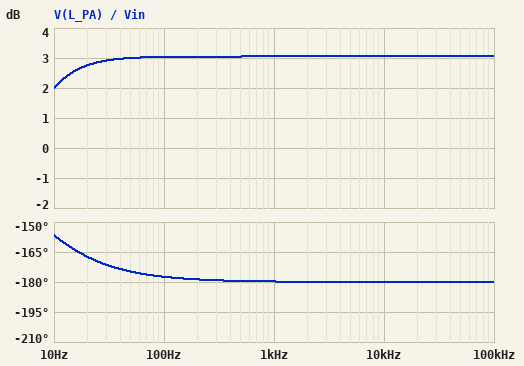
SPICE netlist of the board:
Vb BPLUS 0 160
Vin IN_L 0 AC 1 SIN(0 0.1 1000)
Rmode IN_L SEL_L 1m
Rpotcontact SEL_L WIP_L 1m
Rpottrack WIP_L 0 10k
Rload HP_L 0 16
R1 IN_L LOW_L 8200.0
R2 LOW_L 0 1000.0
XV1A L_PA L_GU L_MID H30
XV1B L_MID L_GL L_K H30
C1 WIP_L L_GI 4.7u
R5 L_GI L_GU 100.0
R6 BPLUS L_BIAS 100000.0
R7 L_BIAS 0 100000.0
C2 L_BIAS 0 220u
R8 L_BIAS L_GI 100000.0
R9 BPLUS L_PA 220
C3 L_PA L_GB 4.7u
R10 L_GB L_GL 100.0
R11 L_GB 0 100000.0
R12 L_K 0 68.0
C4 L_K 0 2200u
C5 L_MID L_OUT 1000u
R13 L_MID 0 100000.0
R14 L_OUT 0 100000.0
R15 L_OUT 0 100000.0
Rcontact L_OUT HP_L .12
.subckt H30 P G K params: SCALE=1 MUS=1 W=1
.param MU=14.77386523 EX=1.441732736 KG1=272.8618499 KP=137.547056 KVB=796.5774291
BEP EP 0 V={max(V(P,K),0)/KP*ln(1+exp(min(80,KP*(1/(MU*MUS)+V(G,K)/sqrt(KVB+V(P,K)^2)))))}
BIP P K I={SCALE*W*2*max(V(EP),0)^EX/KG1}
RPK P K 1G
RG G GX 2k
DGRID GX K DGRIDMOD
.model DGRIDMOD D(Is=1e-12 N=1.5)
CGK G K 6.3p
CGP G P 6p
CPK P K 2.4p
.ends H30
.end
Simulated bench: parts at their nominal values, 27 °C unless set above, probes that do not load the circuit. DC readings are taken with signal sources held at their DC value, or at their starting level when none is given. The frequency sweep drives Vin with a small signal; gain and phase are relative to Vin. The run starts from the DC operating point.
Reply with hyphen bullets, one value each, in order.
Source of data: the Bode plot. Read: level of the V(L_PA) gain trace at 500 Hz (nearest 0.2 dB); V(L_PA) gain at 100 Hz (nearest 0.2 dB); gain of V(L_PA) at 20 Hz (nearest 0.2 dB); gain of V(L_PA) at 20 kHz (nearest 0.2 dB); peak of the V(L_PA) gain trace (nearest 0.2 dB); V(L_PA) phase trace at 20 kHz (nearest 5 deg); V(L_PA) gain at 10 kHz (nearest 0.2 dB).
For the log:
- 3.0 dB
- 3.0 dB
- 2.8 dB
- 3.0 dB
- 3.0 dB
- -180 deg
- 3.0 dB
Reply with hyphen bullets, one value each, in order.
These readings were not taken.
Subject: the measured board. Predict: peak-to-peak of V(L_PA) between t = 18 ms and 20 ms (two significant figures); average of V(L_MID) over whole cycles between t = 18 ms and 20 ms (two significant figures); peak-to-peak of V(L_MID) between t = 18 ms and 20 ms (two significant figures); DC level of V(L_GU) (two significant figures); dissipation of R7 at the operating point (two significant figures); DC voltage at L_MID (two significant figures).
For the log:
- 280 mV
- 82 V
- 93 mV
- 80 V
- 64 mW
- 82 V
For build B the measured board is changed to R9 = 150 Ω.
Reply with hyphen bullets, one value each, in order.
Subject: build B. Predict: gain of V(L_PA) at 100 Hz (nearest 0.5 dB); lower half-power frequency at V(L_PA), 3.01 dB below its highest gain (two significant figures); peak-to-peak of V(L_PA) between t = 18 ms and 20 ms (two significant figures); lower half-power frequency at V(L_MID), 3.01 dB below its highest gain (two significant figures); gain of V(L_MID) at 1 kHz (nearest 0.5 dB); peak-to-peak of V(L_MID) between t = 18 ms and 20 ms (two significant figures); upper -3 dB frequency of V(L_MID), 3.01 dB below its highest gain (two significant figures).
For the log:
- 1.0 dB
- 4.5 Hz
- 230 mV
- 280 mHz
- -7.5 dB
- 83 mV
- 7.8 Hz
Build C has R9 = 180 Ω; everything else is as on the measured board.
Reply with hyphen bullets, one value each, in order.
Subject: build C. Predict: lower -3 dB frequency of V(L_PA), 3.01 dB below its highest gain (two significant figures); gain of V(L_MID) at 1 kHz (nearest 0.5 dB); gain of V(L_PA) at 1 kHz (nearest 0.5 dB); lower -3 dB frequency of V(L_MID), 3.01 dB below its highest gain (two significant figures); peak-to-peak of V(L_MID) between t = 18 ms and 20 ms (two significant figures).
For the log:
- 4.7 Hz
- -7.0 dB
- 2.0 dB
- 280 mHz
- 88 mV
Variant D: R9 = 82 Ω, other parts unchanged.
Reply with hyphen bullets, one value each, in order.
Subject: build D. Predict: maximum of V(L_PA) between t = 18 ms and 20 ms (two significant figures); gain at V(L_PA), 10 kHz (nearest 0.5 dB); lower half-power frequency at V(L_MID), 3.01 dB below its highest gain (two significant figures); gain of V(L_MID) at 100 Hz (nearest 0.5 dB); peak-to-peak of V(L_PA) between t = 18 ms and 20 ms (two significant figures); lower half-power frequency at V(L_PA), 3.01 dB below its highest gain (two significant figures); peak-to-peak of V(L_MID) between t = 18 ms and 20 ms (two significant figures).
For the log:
- 160 V
- -2.5 dB
- 270 mHz
- -9.0 dB
- 150 mV
- 3.7 Hz
- 69 mV
